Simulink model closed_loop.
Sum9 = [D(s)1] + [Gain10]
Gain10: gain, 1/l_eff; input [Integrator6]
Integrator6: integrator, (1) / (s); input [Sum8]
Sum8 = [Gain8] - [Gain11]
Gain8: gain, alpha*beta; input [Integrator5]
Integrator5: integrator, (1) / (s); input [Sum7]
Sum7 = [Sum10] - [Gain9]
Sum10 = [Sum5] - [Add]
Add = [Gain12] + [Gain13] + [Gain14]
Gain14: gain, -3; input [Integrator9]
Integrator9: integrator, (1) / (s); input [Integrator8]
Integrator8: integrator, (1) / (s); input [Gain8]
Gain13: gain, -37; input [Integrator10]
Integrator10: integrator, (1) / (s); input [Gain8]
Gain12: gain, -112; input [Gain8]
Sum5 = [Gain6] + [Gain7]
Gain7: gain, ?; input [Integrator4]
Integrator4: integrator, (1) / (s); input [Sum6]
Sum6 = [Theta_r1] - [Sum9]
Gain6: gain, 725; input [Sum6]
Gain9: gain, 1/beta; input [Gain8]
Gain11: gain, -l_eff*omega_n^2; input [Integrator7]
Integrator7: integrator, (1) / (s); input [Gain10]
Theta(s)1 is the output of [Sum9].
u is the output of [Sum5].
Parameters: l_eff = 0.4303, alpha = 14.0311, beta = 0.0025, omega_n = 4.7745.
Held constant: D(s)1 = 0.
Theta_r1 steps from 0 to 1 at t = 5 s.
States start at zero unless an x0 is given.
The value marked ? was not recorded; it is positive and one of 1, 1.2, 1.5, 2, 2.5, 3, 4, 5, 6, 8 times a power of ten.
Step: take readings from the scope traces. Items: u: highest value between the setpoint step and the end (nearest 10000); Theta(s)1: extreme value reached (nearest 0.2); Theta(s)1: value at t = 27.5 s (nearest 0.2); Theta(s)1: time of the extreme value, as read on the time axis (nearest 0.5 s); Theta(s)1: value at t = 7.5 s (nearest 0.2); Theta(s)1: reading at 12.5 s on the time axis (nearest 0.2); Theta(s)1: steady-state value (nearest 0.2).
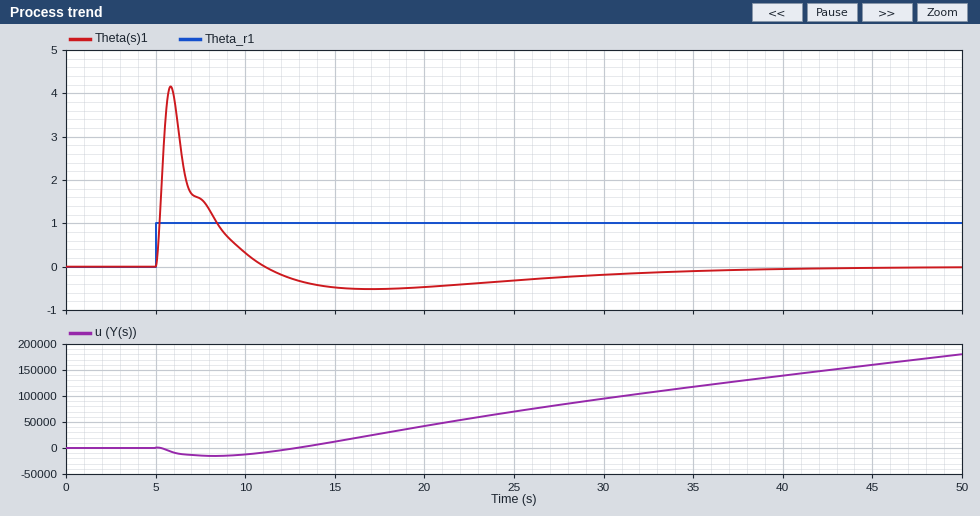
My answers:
180000
4.2
-0.2
6.0 s
1.6
-0.2
0.0
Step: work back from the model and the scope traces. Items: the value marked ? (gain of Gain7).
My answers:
4000
